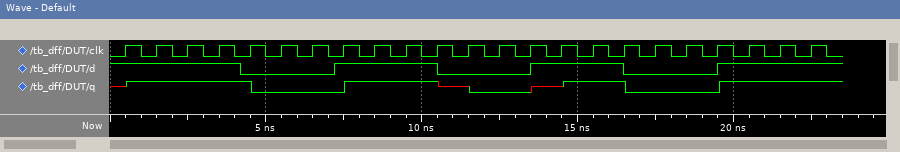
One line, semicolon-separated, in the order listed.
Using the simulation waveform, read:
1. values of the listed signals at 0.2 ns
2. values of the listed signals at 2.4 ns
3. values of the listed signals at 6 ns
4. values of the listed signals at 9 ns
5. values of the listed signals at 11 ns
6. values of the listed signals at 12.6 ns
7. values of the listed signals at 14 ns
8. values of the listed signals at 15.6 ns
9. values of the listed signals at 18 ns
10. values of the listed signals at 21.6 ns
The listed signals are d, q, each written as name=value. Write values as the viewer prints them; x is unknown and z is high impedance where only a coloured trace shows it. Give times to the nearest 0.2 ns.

d=1, q=x; d=1, q=1; d=0, q=0; d=1, q=1; d=0, q=x; d=0, q=0; d=1, q=x; d=1, q=1; d=0, q=0; d=1, q=1
